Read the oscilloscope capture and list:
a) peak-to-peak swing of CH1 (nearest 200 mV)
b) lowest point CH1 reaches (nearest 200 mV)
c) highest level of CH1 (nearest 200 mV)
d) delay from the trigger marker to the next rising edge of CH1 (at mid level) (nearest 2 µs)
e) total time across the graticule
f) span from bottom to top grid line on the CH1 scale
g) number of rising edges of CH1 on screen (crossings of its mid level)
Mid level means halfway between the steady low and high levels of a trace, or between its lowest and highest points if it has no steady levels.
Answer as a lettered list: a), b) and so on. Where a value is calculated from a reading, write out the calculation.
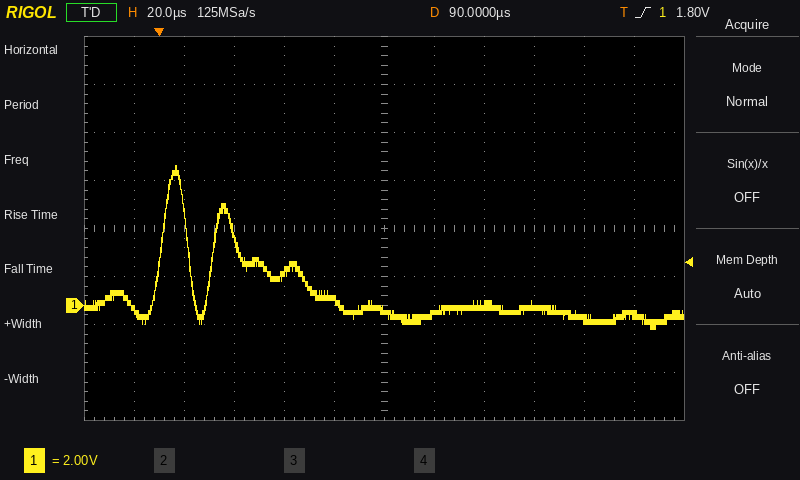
a) 5.8 V − (-1.0 V) = 6.8 V
b) -1.0 V
c) 5.8 V
d) 22 µs
e) 240 µs
f) 16 V
g) 2
